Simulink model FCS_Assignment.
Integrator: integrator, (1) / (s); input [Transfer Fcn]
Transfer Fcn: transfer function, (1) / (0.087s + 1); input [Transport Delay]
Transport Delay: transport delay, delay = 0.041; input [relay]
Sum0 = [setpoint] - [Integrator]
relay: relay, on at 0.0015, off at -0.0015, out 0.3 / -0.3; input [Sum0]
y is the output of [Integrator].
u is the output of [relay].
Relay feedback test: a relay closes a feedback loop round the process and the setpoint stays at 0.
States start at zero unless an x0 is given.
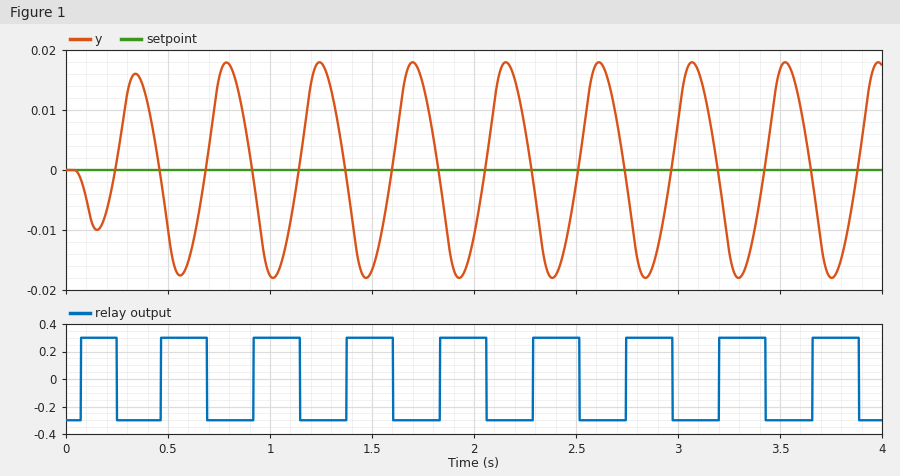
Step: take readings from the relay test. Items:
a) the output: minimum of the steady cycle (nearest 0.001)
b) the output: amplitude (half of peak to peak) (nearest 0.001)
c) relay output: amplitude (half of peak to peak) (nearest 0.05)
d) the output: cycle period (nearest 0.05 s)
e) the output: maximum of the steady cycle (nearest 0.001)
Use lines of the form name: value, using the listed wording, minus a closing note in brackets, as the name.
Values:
the output: minimum of the steady cycle: -0.018
the output: amplitude (half of peak to peak): 0.018
relay output: amplitude (half of peak to peak): 0.30
the output: cycle period: 0.45 s
the output: maximum of the steady cycle: 0.018
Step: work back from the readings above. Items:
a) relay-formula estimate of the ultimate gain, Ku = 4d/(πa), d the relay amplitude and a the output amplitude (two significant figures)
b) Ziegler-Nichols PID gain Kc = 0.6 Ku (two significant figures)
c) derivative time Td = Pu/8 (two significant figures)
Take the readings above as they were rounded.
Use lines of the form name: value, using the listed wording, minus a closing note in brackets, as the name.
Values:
relay-formula estimate of the ultimate gain, Ku = 4d/(πa), d the relay amplitude and a the output amplitude: 21
Ziegler-Nichols PID gain Kc = 0.6 Ku: 13
derivative time Td = Pu/8: 0.056 s
